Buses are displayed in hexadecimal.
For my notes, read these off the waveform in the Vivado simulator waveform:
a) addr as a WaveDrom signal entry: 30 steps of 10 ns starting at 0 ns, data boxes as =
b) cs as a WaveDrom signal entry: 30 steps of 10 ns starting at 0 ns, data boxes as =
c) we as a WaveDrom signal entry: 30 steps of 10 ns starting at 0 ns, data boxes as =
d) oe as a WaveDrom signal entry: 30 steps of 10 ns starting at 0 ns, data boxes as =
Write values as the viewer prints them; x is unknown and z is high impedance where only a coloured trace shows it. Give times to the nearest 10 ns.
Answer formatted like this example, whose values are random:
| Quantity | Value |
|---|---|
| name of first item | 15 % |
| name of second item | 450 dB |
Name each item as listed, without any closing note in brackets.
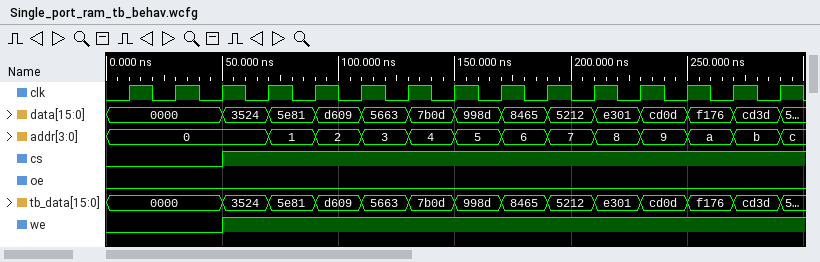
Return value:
| Quantity | Value |
|---|---|
| addr as a WaveDrom signal entry: 30 steps of 10 ns starting at 0 ns, data boxes as = | {name: 'addr', wave: '=......=.=.=.=.=.=.=.=.=.=.=.=', data: '0 1 2 3 4 5 6 7 8 9 a b c'} |
| cs as a WaveDrom signal entry: 30 steps of 10 ns starting at 0 ns, data boxes as = | {name: 'cs', wave: '0....1........................'} |
| we as a WaveDrom signal entry: 30 steps of 10 ns starting at 0 ns, data boxes as = | {name: 'we', wave: '0....1........................'} |
| oe as a WaveDrom signal entry: 30 steps of 10 ns starting at 0 ns, data boxes as = | {name: 'oe', wave: '0.............................'} |
